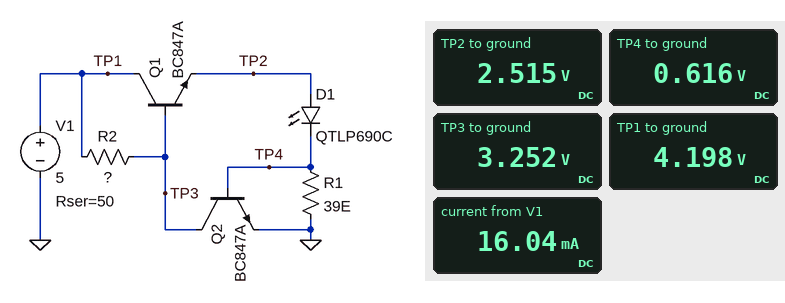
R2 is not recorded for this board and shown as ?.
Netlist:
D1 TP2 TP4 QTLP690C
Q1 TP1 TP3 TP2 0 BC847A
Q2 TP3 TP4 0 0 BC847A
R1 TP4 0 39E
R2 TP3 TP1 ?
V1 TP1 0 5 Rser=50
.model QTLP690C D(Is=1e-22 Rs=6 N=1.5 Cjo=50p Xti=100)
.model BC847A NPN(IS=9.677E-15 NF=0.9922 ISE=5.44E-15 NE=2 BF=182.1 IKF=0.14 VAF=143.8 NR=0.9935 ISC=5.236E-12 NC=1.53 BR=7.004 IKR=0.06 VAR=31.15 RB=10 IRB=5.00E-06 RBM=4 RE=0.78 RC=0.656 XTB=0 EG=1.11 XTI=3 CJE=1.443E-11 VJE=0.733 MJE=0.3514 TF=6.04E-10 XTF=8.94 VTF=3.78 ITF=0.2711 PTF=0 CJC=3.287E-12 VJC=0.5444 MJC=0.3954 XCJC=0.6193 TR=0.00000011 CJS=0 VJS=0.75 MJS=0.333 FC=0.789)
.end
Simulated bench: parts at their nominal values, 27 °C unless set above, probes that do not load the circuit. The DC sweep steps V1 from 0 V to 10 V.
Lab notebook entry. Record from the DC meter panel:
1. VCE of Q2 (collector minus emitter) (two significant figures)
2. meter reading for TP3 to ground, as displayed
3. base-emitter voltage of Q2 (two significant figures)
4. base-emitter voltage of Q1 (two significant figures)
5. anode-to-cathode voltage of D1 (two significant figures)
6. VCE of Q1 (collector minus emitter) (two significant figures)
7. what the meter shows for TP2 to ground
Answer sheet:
3.3 V
3.252 V
620 mV
740 mV
1.9 V
1.7 V
2.515 V
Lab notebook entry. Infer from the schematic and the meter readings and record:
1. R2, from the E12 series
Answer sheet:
2.7 kΩ
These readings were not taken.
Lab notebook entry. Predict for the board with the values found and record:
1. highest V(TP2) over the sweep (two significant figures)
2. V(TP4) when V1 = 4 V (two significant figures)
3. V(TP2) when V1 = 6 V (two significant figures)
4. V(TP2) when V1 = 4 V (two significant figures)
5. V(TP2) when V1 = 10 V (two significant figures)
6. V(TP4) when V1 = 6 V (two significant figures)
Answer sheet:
2.6 V
510 mV
2.5 V
2.4 V
2.6 V
640 mV
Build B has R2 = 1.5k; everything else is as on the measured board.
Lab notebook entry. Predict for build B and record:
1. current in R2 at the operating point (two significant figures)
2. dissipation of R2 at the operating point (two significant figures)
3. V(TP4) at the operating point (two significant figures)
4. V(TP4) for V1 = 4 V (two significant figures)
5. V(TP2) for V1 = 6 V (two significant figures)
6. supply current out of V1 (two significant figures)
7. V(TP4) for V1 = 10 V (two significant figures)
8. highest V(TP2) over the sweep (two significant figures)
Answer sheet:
590 µA
530 µW
630 mV
540 mV
2.6 V
17 mA
690 mV
2.6 V
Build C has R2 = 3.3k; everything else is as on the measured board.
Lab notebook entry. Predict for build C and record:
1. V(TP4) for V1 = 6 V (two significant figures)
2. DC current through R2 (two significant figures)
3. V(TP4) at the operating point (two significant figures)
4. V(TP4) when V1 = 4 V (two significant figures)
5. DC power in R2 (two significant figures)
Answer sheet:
630 mV
290 µA
610 mV
500 mV
280 µW
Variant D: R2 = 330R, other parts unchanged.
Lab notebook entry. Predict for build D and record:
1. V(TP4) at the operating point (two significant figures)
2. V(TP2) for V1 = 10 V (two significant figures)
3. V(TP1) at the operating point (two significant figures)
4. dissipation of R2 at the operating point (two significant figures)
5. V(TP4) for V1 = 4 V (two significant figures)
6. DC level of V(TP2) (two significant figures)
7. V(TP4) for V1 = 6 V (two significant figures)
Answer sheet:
670 mV
2.7 V
4.0 V
1.5 mW
580 mV
2.6 V
690 mV
